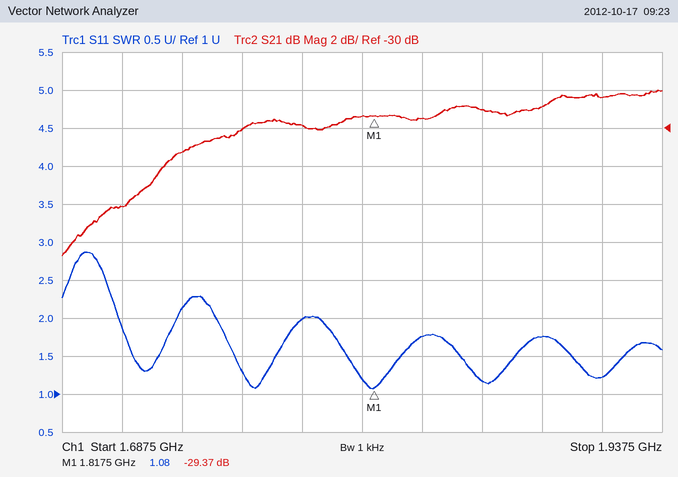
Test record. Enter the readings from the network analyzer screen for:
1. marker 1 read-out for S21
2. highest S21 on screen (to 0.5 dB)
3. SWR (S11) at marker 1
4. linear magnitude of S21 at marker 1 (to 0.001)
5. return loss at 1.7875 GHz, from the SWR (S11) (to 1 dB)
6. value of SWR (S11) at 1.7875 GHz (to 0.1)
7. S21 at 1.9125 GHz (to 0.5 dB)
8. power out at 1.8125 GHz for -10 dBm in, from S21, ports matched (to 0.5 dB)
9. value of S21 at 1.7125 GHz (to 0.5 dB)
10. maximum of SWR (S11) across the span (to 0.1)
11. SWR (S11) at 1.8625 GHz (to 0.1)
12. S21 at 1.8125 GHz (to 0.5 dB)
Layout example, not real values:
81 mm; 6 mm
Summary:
-29.37 dB; -28.0 dB; 1.08; 0.034; 10 dB; 2.0; -28.5 dB; -39.5 dBm; -34.0 dB; 2.9; 1.2; -29.5 dB
